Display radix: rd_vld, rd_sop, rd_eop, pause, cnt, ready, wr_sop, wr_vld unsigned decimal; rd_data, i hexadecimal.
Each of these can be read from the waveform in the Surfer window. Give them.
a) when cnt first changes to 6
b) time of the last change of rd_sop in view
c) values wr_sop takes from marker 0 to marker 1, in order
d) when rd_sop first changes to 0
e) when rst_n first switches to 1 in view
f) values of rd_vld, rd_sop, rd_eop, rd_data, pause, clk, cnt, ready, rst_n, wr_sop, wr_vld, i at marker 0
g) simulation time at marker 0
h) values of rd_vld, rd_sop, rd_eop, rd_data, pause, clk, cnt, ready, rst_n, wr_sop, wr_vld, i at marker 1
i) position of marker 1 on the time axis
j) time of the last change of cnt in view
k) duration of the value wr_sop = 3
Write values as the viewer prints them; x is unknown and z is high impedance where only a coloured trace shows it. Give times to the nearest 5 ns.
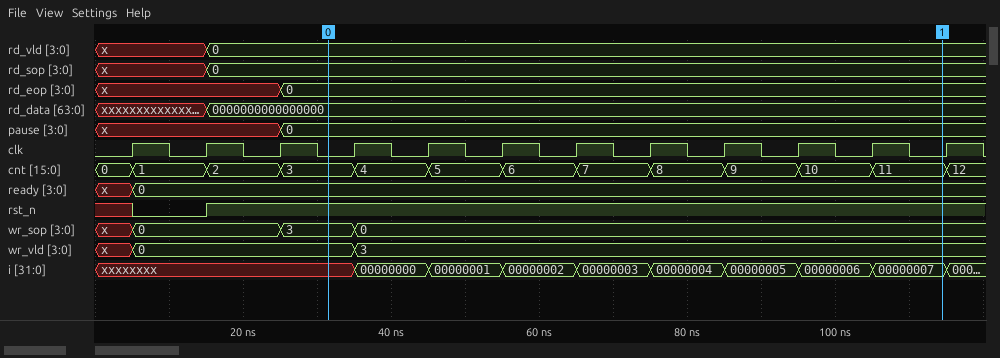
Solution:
55 ns
15 ns
3, 0
15 ns
15 ns
rd_vld=0, rd_sop=0, rd_eop=0, rd_data=0000000000000000, pause=0, clk=0, cnt=3, ready=0, rst_n=1, wr_sop=3, wr_vld=0, i=xxxxxxxx
30 ns
rd_vld=0, rd_sop=0, rd_eop=0, rd_data=0000000000000000, pause=0, clk=0, cnt=11, ready=0, rst_n=1, wr_sop=0, wr_vld=3, i=00000007
115 ns
115 ns
10 ns
